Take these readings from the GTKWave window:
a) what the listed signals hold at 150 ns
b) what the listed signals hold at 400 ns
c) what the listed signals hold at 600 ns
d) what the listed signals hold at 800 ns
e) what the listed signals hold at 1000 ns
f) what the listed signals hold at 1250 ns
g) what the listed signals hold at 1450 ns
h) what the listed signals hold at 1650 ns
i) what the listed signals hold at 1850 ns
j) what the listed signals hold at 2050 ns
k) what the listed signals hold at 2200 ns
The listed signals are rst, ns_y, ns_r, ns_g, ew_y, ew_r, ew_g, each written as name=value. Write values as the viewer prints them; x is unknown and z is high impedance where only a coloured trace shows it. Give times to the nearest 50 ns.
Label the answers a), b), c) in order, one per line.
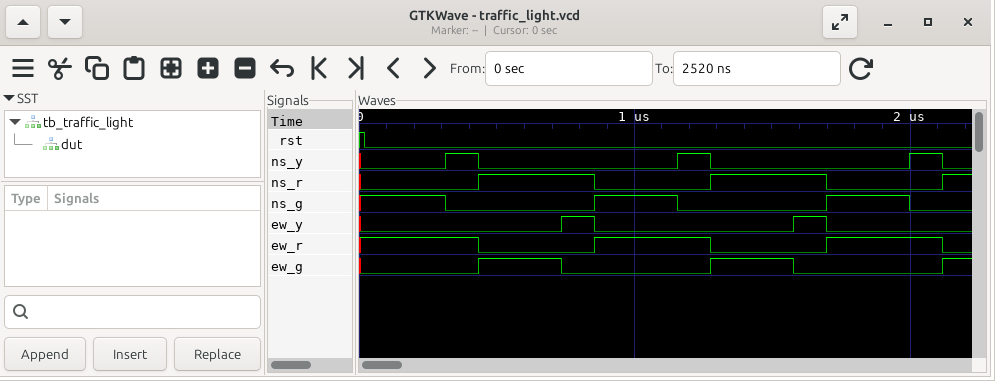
a) rst=0, ns_y=0, ns_r=0, ns_g=1, ew_y=0, ew_r=1, ew_g=0
b) rst=0, ns_y=1, ns_r=0, ns_g=0, ew_y=0, ew_r=1, ew_g=0
c) rst=0, ns_y=0, ns_r=1, ns_g=0, ew_y=0, ew_r=0, ew_g=1
d) rst=0, ns_y=0, ns_r=1, ns_g=0, ew_y=1, ew_r=0, ew_g=0
e) rst=0, ns_y=0, ns_r=0, ns_g=1, ew_y=0, ew_r=1, ew_g=0
f) rst=0, ns_y=1, ns_r=0, ns_g=0, ew_y=0, ew_r=1, ew_g=0
g) rst=0, ns_y=0, ns_r=1, ns_g=0, ew_y=0, ew_r=0, ew_g=1
h) rst=0, ns_y=0, ns_r=1, ns_g=0, ew_y=1, ew_r=0, ew_g=0
i) rst=0, ns_y=0, ns_r=0, ns_g=1, ew_y=0, ew_r=1, ew_g=0
j) rst=0, ns_y=1, ns_r=0, ns_g=0, ew_y=0, ew_r=1, ew_g=0
k) rst=0, ns_y=0, ns_r=1, ns_g=0, ew_y=0, ew_r=0, ew_g=1
